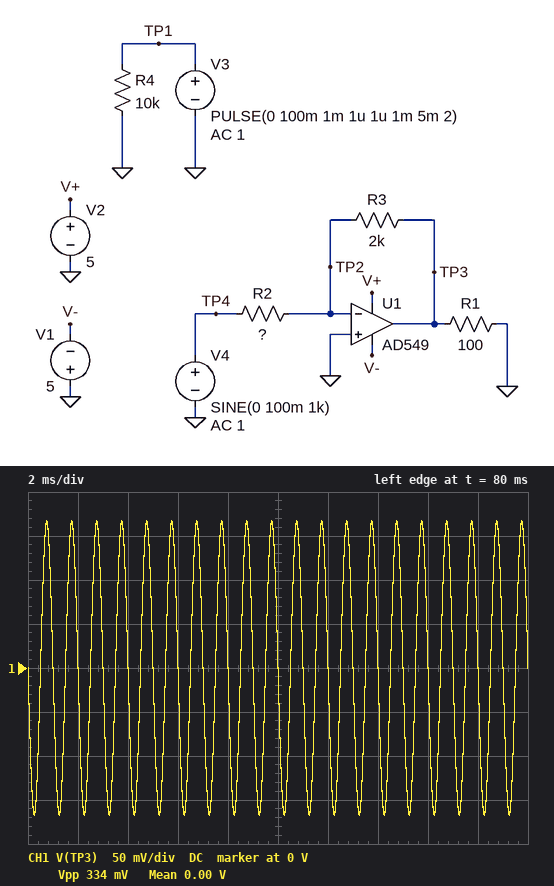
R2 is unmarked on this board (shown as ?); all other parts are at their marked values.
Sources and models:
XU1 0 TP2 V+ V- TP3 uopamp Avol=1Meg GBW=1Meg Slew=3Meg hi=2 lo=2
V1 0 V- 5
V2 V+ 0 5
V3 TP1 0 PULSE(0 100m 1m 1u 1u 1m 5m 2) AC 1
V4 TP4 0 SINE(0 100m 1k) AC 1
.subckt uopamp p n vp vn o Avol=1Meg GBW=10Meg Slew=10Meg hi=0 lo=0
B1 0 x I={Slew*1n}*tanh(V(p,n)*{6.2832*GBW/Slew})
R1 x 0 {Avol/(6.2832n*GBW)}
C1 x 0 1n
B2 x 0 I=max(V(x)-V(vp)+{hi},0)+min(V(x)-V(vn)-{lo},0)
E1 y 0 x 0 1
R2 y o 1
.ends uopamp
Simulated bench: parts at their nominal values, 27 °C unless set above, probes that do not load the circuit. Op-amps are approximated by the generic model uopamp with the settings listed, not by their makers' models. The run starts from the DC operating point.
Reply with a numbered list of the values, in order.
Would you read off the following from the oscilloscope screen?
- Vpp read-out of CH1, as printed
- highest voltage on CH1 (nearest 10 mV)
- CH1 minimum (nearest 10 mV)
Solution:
1. 334 mV
2. 170 mV
3. -170 mV
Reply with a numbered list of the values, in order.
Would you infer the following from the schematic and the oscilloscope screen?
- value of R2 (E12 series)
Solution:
1. 1.2 kΩ
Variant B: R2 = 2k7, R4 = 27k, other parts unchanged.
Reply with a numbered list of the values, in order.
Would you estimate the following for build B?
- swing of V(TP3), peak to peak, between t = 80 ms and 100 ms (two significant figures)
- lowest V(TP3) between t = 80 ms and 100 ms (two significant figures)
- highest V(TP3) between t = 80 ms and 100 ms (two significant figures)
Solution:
1. 150 mV
2. -74 mV
3. 74 mV
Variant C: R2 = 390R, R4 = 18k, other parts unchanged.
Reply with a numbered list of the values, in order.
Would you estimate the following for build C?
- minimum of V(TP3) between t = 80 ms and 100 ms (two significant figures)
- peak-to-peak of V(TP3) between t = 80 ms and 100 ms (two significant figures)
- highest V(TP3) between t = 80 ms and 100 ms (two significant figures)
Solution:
1. -510 mV
2. 1.0 V
3. 510 mV
